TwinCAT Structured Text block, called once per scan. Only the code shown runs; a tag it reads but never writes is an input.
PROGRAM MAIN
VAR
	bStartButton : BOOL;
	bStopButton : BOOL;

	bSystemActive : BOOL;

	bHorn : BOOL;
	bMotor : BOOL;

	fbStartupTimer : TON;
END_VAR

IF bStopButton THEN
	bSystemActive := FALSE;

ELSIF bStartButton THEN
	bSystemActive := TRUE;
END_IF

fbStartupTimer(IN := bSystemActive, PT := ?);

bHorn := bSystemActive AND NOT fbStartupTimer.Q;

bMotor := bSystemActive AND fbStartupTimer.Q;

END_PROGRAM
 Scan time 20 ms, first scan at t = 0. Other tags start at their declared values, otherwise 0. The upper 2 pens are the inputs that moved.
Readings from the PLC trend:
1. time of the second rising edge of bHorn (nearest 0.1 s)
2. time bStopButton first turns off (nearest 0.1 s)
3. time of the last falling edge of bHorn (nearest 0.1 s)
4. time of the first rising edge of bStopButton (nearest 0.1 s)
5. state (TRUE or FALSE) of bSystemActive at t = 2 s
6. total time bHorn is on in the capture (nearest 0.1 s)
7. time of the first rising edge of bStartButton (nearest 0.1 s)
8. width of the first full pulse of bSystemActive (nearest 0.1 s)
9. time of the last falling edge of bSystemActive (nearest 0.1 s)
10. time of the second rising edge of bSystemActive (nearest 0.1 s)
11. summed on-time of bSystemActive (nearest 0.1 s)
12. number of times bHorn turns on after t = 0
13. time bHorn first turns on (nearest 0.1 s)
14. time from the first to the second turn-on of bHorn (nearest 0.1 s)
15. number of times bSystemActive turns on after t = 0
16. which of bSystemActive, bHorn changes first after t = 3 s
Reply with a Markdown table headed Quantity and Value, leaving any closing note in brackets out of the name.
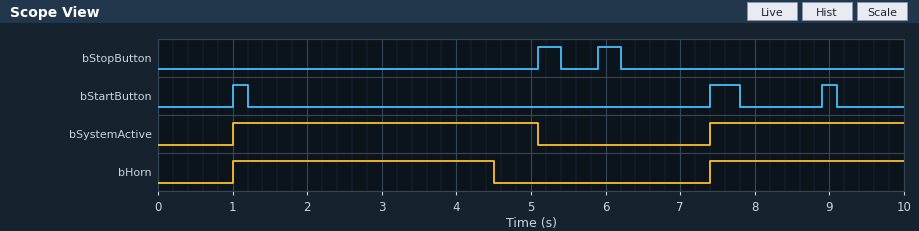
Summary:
| Quantity | Value |
|---|---|
| time of the second rising edge of bHorn | 7.4 s |
| time bStopButton first turns off | 5.4 s |
| time of the last falling edge of bHorn | 4.5 s |
| time of the first rising edge of bStopButton | 5.1 s |
| state (TRUE or FALSE) of bSystemActive at t = 2 s | TRUE |
| total time bHorn is on in the capture | 6.1 s |
| time of the first rising edge of bStartButton | 1.0 s |
| width of the first full pulse of bSystemActive | 4.1 s |
| time of the last falling edge of bSystemActive | 5.1 s |
| time of the second rising edge of bSystemActive | 7.4 s |
| summed on-time of bSystemActive | 6.7 s |
| number of times bHorn turns on after t = 0 | 2 |
| time bHorn first turns on | 1.0 s |
| time from the first to the second turn-on of bHorn | 6.4 s |
| number of times bSystemActive turns on after t = 0 | 2 |
| which of bSystemActive, bHorn changes first after t = 3 s | bHorn |
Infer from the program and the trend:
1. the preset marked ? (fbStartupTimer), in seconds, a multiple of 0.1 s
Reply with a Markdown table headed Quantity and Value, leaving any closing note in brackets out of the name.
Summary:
| Quantity | Value |
|---|---|
| the preset marked ? (fbStartupTimer), in seconds, a multiple of 0.1 s | 3.5 s |
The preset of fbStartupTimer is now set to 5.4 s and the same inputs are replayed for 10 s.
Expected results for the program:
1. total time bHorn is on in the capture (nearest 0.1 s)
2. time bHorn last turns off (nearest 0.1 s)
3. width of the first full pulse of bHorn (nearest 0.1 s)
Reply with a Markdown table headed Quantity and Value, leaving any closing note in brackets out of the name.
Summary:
| Quantity | Value |
|---|---|
| total time bHorn is on in the capture | 6.7 s |
| time bHorn last turns off | 5.1 s |
| width of the first full pulse of bHorn | 4.1 s |
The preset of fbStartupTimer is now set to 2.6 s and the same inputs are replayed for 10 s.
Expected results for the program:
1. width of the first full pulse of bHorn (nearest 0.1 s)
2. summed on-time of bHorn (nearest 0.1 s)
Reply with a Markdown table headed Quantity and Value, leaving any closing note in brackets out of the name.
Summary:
| Quantity | Value |
|---|---|
| width of the first full pulse of bHorn | 2.6 s |
| summed on-time of bHorn | 5.2 s |
